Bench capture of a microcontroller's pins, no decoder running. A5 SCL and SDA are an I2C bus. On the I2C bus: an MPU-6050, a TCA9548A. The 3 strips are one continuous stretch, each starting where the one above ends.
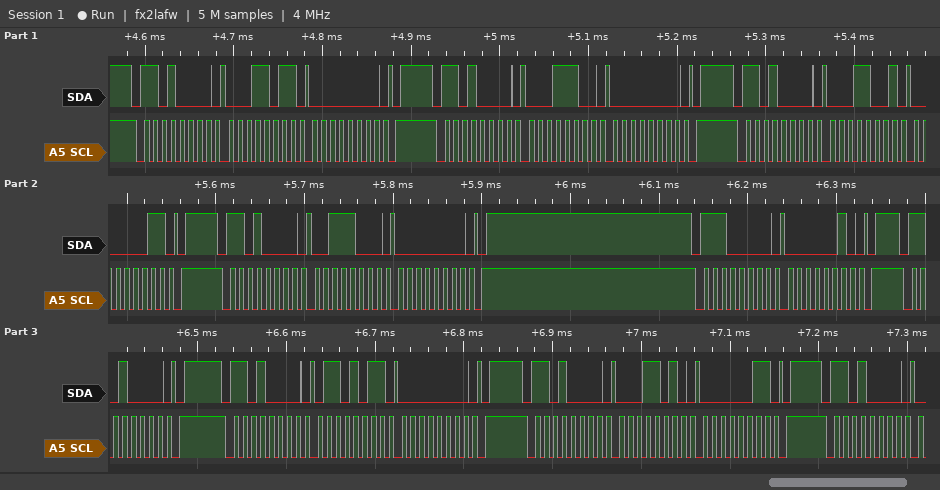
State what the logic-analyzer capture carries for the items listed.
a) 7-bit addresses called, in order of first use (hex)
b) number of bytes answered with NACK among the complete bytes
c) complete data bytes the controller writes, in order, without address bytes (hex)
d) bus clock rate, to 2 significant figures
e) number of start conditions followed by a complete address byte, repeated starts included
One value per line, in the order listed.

0x68 0x70
0
1B 00 1C 00 19 03 38 00 02 6B 00 1A 03
100 kHz
9
